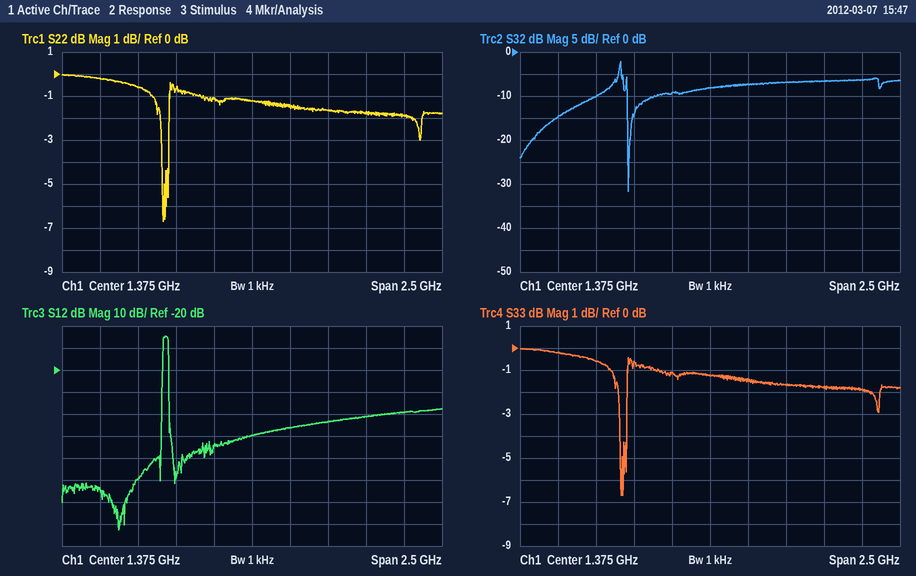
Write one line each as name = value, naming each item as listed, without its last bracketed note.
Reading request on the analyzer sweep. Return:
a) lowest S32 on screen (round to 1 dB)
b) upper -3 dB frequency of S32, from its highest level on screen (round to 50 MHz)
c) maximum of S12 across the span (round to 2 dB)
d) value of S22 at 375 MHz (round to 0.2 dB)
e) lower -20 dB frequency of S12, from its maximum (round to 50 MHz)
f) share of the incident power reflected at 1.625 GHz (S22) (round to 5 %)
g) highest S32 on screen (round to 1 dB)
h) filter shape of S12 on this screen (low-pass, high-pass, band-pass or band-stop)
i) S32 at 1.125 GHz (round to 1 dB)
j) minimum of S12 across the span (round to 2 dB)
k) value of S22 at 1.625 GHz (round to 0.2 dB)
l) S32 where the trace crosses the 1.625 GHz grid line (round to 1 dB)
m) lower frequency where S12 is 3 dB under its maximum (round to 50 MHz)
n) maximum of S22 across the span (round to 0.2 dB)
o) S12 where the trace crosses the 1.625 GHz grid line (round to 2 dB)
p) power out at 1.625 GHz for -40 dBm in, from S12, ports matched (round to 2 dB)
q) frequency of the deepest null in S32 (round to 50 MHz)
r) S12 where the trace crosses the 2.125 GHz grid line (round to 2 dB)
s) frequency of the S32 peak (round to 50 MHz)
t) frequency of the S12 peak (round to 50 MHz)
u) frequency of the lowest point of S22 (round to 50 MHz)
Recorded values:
lowest S32 on screen = -32 dB
upper -3 dB frequency of S32, from its highest level on screen = 800 MHz
maximum of S12 across the span = -4 dB
value of S22 at 375 MHz = -0.2 dB
lower -20 dB frequency of S12, from its maximum = 800 MHz
share of the incident power reflected at 1.625 GHz (S22) = 70 %
highest S32 on screen = -2 dB
filter shape of S12 on this screen = band-pass
S32 at 1.125 GHz = -9 dB
minimum of S12 across the span = -92 dB
value of S22 at 1.625 GHz = -1.4 dB
S32 where the trace crosses the 1.625 GHz grid line = -7 dB
lower frequency where S12 is 3 dB under its maximum = 800 MHz
maximum of S22 across the span = 0.0 dB
S12 where the trace crosses the 1.625 GHz grid line = -46 dB
power out at 1.625 GHz for -40 dBm in, from S12, ports matched = -86 dBm
frequency of the deepest null in S32 = 850 MHz
S12 where the trace crosses the 2.125 GHz grid line = -42 dB
frequency of the S32 peak = 800 MHz
frequency of the S12 peak = 800 MHz
frequency of the lowest point of S22 = 800 MHz
